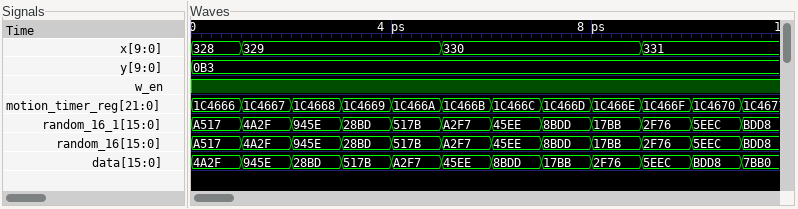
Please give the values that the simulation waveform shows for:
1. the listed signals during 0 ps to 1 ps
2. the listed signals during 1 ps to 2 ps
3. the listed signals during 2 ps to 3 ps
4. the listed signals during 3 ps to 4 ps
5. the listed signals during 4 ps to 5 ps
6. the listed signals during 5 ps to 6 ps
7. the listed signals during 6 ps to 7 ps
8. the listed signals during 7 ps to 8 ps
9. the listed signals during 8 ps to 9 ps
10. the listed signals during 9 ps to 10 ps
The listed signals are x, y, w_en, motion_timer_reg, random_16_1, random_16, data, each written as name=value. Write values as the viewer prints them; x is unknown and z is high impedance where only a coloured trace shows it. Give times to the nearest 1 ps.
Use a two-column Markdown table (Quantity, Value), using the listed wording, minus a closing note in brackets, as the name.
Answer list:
| Quantity | Value |
|---|---|
| the listed signals during 0 ps to 1 ps | x=328, y=0B3, w_en=1, motion_timer_reg=1C4666, random_16_1=A517, random_16=A517, data=4A2F |
| the listed signals during 1 ps to 2 ps | x=329, y=0B3, w_en=1, motion_timer_reg=1C4667, random_16_1=4A2F, random_16=4A2F, data=945E |
| the listed signals during 2 ps to 3 ps | x=329, y=0B3, w_en=1, motion_timer_reg=1C4668, random_16_1=945E, random_16=945E, data=28BD |
| the listed signals during 3 ps to 4 ps | x=329, y=0B3, w_en=1, motion_timer_reg=1C4669, random_16_1=28BD, random_16=28BD, data=517B |
| the listed signals during 4 ps to 5 ps | x=329, y=0B3, w_en=1, motion_timer_reg=1C466A, random_16_1=517B, random_16=517B, data=A2F7 |
| the listed signals during 5 ps to 6 ps | x=330, y=0B3, w_en=1, motion_timer_reg=1C466B, random_16_1=A2F7, random_16=A2F7, data=45EE |
| the listed signals during 6 ps to 7 ps | x=330, y=0B3, w_en=1, motion_timer_reg=1C466C, random_16_1=45EE, random_16=45EE, data=8BDD |
| the listed signals during 7 ps to 8 ps | x=330, y=0B3, w_en=1, motion_timer_reg=1C466D, random_16_1=8BDD, random_16=8BDD, data=17BB |
| the listed signals during 8 ps to 9 ps | x=330, y=0B3, w_en=1, motion_timer_reg=1C466E, random_16_1=17BB, random_16=17BB, data=2F76 |
| the listed signals during 9 ps to 10 ps | x=331, y=0B3, w_en=1, motion_timer_reg=1C466F, random_16_1=2F76, random_16=2F76, data=5EEC |
